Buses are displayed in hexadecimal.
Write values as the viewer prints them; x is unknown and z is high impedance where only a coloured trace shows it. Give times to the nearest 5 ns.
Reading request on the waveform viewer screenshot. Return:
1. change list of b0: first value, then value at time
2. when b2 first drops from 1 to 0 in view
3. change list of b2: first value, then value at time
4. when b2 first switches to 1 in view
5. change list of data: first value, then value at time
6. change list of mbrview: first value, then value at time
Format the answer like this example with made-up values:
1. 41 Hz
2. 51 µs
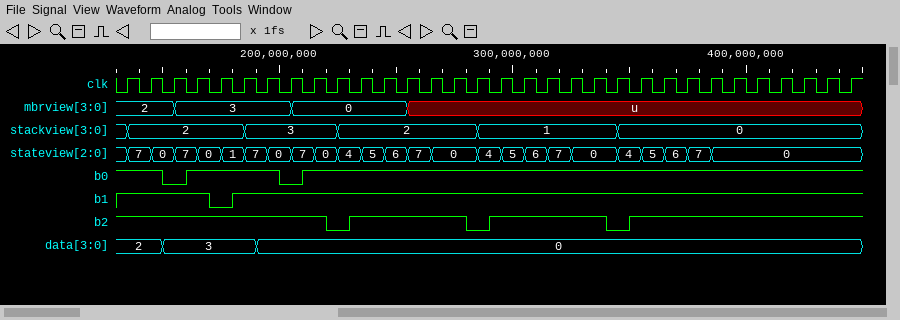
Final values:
1. 1, 0 at 150 ns, 1 at 160 ns, 0 at 200 ns, 1 at 210 ns
2. 220 ns
3. 1, 0 at 220 ns, 1 at 230 ns, 0 at 280 ns, 1 at 290 ns, 0 at 340 ns, 1 at 350 ns
4. 230 ns
5. 2, 3 at 150 ns, 0 at 190 ns
6. 2, 3 at 155 ns, 0 at 205 ns, u at 255 ns
